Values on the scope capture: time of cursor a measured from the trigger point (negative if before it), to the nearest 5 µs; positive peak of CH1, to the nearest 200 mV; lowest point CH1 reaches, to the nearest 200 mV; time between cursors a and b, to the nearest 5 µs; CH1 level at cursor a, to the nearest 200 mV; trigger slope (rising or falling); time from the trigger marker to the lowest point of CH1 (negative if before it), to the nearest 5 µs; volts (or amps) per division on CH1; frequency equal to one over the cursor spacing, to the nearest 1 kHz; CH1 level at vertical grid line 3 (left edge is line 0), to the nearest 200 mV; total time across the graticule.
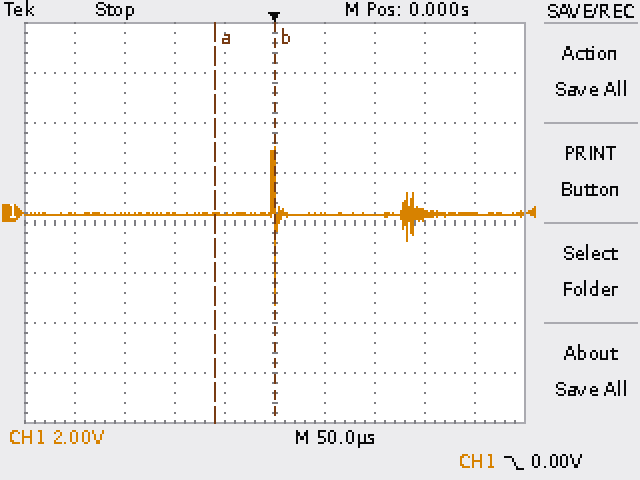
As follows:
-60 µs
2.6 V
-3.6 V
60 µs
0.0 V
falling
0 µs
2 V
17 kHz
0.0 V
500 µs
